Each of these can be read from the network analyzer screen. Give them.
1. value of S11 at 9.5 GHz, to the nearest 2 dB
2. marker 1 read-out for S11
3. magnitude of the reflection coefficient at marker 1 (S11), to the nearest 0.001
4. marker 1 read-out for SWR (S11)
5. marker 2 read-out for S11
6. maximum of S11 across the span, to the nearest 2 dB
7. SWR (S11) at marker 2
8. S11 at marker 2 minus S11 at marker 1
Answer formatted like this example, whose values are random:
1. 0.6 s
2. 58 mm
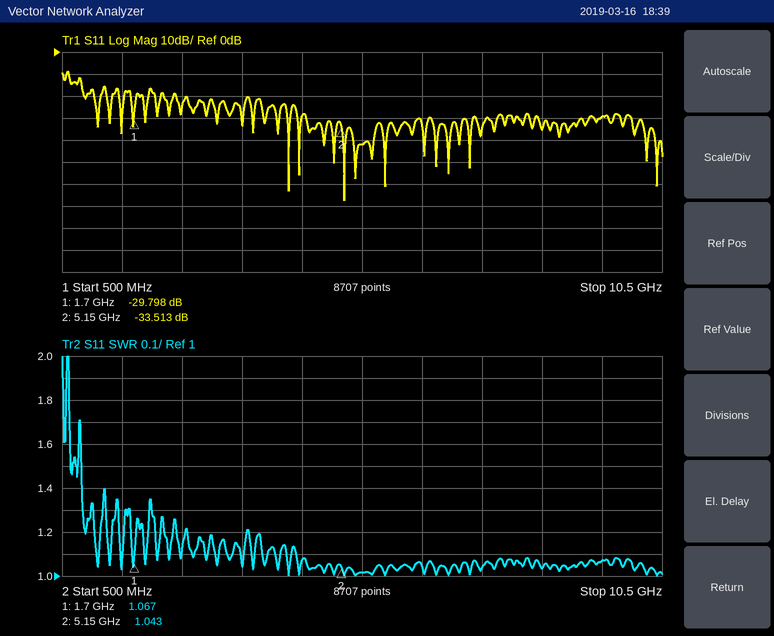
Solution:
1. -30 dB
2. -29.798 dB
3. 0.032
4. 1.067
5. -33.513 dB
6. -8 dB
7. 1.043
8. -3.715 dB
